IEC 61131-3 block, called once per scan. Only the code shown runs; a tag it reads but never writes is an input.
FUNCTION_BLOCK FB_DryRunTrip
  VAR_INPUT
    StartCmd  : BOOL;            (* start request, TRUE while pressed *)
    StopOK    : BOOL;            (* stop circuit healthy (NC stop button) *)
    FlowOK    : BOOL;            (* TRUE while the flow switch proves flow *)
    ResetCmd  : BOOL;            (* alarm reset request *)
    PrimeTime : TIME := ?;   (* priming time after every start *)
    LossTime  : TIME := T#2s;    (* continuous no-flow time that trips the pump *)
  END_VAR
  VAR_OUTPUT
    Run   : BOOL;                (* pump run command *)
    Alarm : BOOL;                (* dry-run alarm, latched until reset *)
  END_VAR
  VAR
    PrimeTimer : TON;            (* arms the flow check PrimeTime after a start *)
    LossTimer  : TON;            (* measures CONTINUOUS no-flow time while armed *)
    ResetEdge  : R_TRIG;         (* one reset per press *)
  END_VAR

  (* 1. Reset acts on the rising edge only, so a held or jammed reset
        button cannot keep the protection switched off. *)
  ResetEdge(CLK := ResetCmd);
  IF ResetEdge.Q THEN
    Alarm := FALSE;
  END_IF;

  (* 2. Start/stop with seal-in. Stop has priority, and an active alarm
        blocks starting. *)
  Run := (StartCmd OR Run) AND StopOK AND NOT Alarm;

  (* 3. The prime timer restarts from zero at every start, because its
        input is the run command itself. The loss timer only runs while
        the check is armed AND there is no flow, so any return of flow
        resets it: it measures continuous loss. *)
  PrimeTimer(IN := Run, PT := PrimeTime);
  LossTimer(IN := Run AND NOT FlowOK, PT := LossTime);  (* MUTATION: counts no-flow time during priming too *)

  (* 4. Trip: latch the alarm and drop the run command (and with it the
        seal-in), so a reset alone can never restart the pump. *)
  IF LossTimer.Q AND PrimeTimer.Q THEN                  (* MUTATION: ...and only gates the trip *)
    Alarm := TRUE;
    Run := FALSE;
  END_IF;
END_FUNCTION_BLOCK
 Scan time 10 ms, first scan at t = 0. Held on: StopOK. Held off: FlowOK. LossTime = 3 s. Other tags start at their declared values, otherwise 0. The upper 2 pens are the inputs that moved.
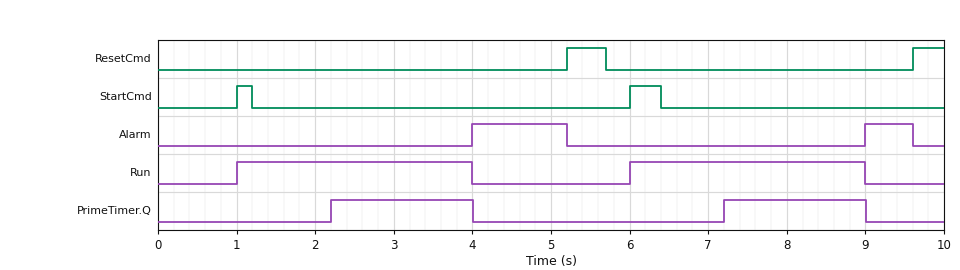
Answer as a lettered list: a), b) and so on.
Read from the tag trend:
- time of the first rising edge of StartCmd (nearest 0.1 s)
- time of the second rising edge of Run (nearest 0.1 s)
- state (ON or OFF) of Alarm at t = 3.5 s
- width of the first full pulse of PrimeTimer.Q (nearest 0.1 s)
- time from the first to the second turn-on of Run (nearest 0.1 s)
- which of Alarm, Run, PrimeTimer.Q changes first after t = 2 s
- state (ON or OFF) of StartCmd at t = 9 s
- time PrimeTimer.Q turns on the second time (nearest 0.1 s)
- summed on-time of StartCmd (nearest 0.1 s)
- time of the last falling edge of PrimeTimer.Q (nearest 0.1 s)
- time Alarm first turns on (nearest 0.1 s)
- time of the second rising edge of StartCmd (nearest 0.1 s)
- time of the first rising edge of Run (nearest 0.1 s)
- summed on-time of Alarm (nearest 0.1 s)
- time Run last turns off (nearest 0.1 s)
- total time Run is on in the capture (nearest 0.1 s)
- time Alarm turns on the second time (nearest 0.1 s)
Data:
a) 1.0 s
b) 6.0 s
c) OFF
d) 1.8 s
e) 5.0 s
f) PrimeTimer.Q
g) OFF
h) 7.2 s
i) 0.6 s
j) 9.0 s
k) 4.0 s
l) 6.0 s
m) 1.0 s
n) 1.8 s
o) 9.0 s
p) 6.0 s
q) 9.0 s
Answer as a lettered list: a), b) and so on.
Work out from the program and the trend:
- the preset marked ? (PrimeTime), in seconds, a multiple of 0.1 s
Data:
a) 1.2 s
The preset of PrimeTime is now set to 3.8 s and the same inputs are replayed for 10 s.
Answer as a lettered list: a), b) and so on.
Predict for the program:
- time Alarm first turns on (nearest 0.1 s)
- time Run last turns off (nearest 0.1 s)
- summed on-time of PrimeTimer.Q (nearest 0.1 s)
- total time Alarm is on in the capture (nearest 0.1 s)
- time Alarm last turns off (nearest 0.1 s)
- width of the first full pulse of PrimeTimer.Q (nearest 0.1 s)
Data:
a) 4.8 s
b) 9.8 s
c) 0.0 s
d) 0.6 s
e) 5.2 s
f) 0.0 s
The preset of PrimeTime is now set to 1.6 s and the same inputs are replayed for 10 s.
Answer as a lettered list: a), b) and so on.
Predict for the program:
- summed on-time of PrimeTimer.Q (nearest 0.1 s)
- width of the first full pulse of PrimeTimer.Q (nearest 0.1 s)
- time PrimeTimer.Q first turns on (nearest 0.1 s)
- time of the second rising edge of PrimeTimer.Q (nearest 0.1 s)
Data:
a) 2.8 s
b) 1.4 s
c) 2.6 s
d) 7.6 s
